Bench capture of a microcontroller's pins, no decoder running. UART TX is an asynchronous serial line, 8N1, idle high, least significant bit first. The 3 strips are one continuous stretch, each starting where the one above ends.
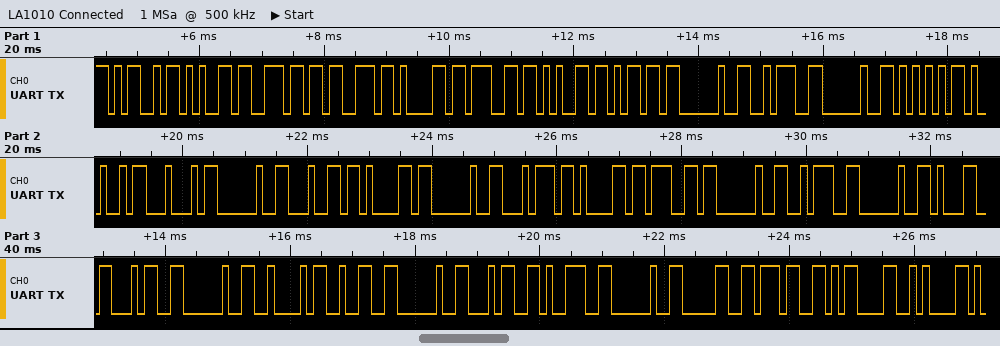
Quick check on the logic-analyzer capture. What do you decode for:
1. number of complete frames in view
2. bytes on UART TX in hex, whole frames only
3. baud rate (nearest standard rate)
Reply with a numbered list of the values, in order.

1. 37
2. 4D 65 6E 73 61 67 65 6D 20 3A 20 55 49 44 20 64 61 20 74 61 67 20 3A 20 31 34 20 42 32 20 34 39 20 30 37 0D 0A
3. 9600 baud
